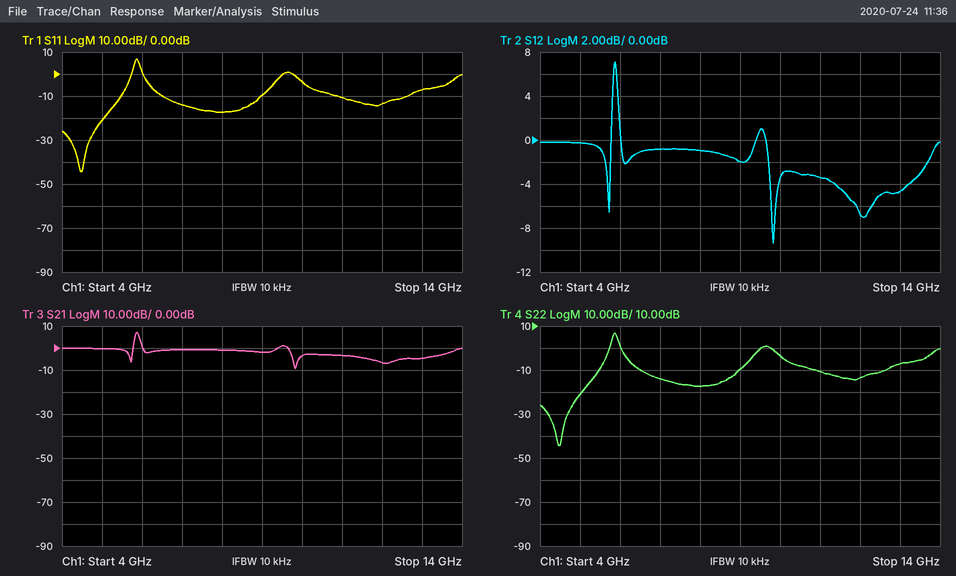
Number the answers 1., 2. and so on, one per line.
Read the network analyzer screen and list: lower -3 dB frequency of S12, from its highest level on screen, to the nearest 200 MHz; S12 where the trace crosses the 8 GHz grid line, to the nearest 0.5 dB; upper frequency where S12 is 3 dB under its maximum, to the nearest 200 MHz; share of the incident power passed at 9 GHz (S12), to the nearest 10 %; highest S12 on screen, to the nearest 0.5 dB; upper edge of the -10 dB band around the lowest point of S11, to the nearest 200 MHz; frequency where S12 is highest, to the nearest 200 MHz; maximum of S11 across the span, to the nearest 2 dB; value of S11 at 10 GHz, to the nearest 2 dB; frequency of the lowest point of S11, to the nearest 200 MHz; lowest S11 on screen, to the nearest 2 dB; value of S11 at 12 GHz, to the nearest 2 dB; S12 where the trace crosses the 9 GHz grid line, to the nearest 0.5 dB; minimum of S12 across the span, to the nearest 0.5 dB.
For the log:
1. 5.8 GHz
2. -1.0 dB
3. 6.0 GHz
4. 60 %
5. 7.0 dB
6. 5.4 GHz
7. 5.8 GHz
8. 6 dB
9. -4 dB
10. 4.4 GHz
11. -44 dB
12. -14 dB
13. -2.0 dB
14. -9.5 dB
